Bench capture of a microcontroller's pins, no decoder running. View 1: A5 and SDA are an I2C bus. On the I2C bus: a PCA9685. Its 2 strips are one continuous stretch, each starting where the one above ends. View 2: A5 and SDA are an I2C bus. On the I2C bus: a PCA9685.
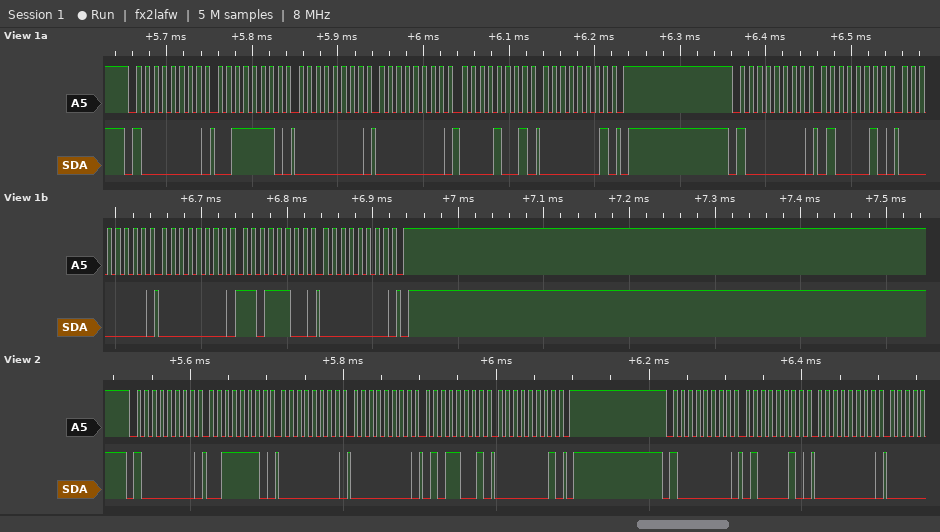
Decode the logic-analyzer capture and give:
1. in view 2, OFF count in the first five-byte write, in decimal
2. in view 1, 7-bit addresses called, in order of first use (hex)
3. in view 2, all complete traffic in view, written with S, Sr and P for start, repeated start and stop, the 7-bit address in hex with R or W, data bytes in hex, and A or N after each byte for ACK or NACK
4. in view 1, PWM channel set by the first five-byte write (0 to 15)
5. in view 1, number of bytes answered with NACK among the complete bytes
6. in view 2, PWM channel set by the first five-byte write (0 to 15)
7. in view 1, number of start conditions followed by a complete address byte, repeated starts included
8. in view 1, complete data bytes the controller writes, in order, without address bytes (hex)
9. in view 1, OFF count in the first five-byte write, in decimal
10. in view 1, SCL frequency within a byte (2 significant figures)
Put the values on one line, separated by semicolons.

345; 0x40; S 40W A 3E A 00 A 00 A 59 A 01 A P S 40W A 42 A 00 A; 14; 0; 14; 2; 3E 00 00 09 01 42 00 00 DC 00; 265; 100 kHz
